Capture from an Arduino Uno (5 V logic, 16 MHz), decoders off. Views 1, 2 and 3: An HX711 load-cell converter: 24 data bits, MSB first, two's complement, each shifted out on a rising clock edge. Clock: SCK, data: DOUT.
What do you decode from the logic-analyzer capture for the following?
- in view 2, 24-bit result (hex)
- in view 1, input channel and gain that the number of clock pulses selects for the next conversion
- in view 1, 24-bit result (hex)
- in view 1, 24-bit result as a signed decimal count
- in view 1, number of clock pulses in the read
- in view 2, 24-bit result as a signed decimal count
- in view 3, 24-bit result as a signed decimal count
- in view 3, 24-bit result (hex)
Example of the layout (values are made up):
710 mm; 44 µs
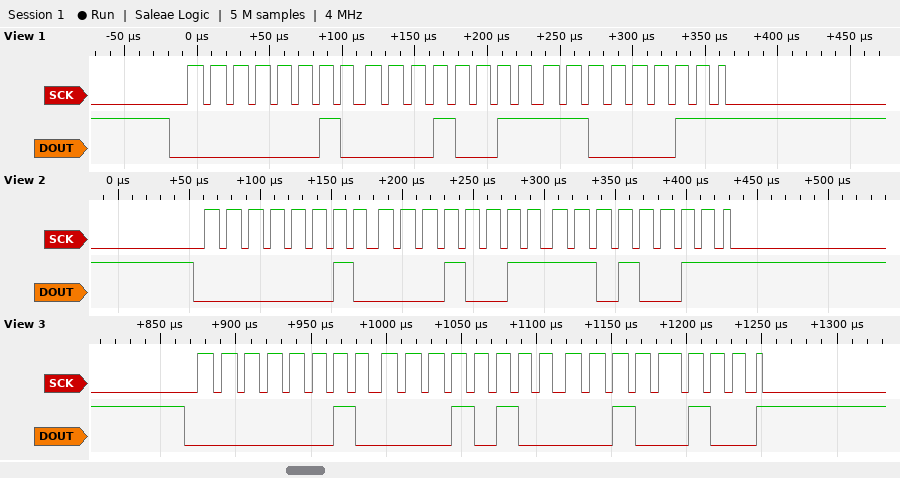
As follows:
0x0213D3; channel A, gain 128; 0x0213C3; 136131; 25; 136147; 136228; 0x021424
